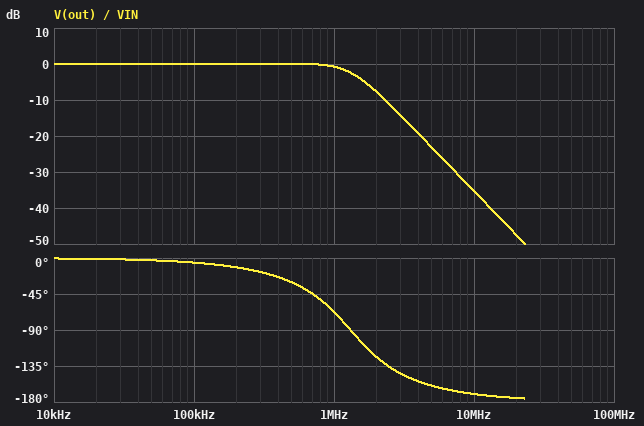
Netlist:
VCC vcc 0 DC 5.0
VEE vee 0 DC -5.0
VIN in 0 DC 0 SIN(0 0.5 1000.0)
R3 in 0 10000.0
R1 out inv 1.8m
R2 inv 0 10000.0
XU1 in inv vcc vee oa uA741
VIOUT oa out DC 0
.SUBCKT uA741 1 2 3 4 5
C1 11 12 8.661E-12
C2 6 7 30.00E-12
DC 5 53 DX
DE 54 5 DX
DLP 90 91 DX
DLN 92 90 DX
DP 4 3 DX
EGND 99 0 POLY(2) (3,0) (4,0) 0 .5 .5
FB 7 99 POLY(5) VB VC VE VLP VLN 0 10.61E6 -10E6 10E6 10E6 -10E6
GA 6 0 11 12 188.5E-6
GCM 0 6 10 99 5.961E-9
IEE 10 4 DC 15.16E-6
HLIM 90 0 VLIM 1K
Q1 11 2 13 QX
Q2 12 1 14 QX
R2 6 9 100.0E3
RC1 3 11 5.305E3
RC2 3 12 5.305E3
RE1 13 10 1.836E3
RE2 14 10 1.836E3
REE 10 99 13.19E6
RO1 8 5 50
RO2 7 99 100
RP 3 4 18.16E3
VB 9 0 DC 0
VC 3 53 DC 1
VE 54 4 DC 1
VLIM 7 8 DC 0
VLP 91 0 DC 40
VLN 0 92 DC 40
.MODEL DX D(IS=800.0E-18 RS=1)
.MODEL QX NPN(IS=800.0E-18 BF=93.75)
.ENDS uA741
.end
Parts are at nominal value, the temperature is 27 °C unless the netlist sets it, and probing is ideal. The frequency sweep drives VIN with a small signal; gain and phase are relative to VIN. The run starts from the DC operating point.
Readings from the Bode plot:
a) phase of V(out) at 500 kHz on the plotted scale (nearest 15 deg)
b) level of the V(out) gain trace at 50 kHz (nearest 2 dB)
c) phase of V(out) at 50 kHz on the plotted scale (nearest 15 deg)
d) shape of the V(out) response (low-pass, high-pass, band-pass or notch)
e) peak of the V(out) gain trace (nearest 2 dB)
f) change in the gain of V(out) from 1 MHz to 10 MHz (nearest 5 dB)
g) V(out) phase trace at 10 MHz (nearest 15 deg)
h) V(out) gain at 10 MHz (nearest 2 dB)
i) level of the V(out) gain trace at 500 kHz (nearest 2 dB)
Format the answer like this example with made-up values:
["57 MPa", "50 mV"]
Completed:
["-30 deg", "0 dB", "0 deg", "low-pass", "0 dB", "-35 dB", "-165 deg", "-36 dB", "0 dB"]
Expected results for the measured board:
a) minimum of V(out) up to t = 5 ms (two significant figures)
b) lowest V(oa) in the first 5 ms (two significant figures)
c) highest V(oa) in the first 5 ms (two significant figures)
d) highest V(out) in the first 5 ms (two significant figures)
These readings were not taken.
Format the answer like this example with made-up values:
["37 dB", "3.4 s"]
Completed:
["-500 mV", "-500 mV", "500 mV", "500 mV"]
